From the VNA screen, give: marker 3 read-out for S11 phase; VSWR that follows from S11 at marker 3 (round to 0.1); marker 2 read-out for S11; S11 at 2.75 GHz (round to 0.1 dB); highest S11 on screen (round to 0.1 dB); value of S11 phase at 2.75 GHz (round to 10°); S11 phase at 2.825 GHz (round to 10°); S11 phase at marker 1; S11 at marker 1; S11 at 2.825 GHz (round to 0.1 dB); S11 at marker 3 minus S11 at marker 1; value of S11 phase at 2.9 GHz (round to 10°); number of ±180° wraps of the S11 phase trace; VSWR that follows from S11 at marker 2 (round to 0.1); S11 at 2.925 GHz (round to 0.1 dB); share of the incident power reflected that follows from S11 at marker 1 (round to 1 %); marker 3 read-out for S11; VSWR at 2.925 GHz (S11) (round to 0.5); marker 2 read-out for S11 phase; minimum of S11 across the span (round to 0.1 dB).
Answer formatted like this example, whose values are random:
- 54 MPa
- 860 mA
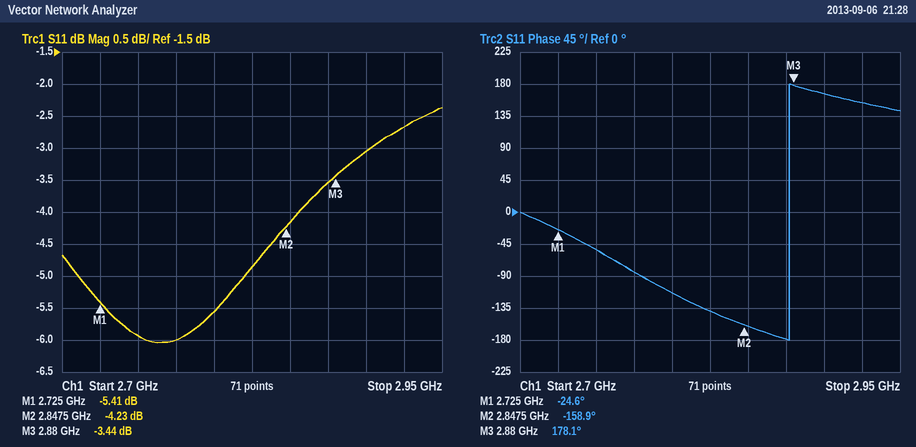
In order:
- 178.1°
- 5.1
- -4.23 dB
- -5.9 dB
- -2.4 dB
- -50°
- -140°
- -24.6°
- -5.41 dB
- -4.9 dB
- 1.97 dB
- 170°
- 1
- 4.2
- -2.7 dB
- 29 %
- -3.44 dB
- 6.5
- -158.9°
- -6.0 dB
